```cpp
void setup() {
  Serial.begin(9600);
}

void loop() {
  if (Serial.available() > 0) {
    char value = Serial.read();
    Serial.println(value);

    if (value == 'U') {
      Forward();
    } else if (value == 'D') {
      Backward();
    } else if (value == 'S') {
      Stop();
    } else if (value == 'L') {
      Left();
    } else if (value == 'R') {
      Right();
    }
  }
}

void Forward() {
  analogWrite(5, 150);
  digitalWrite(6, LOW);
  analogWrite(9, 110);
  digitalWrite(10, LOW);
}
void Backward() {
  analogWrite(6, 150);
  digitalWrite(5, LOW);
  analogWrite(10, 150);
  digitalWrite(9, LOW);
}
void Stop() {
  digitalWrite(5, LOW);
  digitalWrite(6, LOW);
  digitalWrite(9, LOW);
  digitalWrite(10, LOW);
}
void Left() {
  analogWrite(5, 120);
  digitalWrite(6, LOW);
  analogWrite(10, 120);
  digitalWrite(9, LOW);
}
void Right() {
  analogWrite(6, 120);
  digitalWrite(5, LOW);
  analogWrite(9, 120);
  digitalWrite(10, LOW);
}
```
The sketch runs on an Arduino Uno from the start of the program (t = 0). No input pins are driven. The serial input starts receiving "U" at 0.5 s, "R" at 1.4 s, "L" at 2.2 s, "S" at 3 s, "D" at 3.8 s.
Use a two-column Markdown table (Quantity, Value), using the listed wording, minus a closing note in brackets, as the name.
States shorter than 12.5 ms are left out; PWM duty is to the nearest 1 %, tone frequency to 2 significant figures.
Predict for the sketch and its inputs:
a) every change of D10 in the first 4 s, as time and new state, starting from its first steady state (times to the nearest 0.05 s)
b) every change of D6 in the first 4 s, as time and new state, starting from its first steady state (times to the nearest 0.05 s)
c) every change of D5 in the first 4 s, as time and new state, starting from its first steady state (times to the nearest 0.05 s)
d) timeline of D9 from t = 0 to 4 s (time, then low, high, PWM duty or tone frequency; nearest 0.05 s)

| Quantity | Value |
|---|---|
| every change of D10 in the first 4 s, as time and new state, starting from its first steady state | 2.2 s PWM 47 %; 3 s low; 3.8 s PWM 59 % |
| every change of D6 in the first 4 s, as time and new state, starting from its first steady state | 1.4 s PWM 47 %; 2.2 s low; 3.8 s PWM 59 % |
| every change of D5 in the first 4 s, as time and new state, starting from its first steady state | 0.5 s PWM 59 %; 1.4 s low; 2.2 s PWM 47 %; 3 s low |
| timeline of D9 from t = 0 to 4 s | 0.5 s PWM 43 %; 1.4 s PWM 47 %; 2.2 s low |
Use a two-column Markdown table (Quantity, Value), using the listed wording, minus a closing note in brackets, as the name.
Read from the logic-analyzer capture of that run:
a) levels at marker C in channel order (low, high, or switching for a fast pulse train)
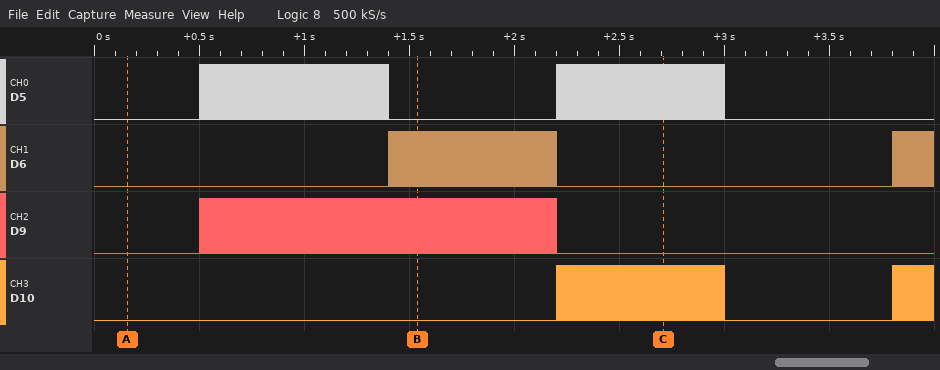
| Quantity | Value |
|---|---|
| levels at marker C in channel order | D5 switching, D6 low, D9 low, D10 switching |
